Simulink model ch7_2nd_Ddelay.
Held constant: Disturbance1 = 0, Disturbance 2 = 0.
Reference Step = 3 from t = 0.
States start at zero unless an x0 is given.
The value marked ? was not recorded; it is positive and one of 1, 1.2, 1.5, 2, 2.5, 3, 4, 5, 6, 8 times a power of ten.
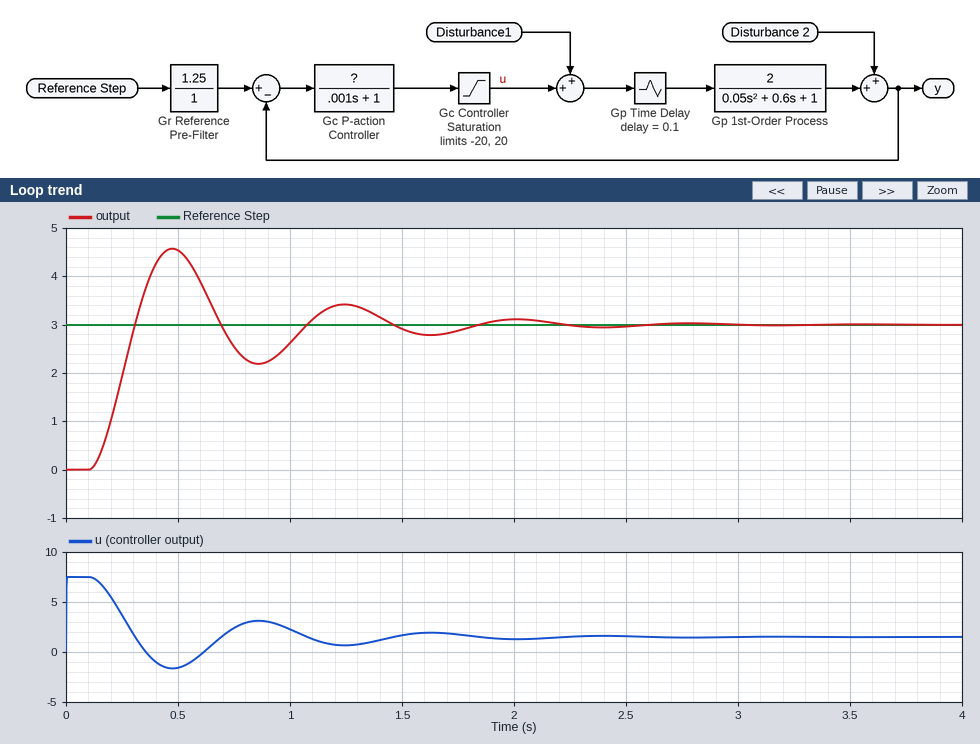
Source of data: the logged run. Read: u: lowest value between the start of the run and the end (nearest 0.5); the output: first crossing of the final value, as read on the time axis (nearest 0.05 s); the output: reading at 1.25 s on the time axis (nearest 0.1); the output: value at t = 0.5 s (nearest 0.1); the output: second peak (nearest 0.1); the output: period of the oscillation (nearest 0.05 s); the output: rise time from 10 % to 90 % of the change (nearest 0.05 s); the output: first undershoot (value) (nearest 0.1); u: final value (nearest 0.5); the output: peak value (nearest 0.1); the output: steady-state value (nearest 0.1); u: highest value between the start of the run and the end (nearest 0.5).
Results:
-1.5
0.30 s
3.4
4.5
3.4
0.75 s
0.15 s
2.2
1.5
4.6
3.0
7.5
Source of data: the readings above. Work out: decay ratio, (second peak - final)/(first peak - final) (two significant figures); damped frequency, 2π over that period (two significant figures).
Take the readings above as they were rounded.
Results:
0.25
8.4 rad/s
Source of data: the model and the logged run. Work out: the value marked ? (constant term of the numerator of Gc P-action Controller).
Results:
2
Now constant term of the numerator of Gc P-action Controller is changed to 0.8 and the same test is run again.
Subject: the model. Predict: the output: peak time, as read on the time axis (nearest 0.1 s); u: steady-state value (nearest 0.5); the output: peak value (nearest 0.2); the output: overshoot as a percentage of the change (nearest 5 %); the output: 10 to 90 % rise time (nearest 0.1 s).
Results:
0.7 s
1.0
2.6
10 %
0.3 s
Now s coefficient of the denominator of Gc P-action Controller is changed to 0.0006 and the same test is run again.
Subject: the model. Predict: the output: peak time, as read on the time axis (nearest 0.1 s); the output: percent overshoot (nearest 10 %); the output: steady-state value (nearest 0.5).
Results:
0.5 s
50 %
3.0
